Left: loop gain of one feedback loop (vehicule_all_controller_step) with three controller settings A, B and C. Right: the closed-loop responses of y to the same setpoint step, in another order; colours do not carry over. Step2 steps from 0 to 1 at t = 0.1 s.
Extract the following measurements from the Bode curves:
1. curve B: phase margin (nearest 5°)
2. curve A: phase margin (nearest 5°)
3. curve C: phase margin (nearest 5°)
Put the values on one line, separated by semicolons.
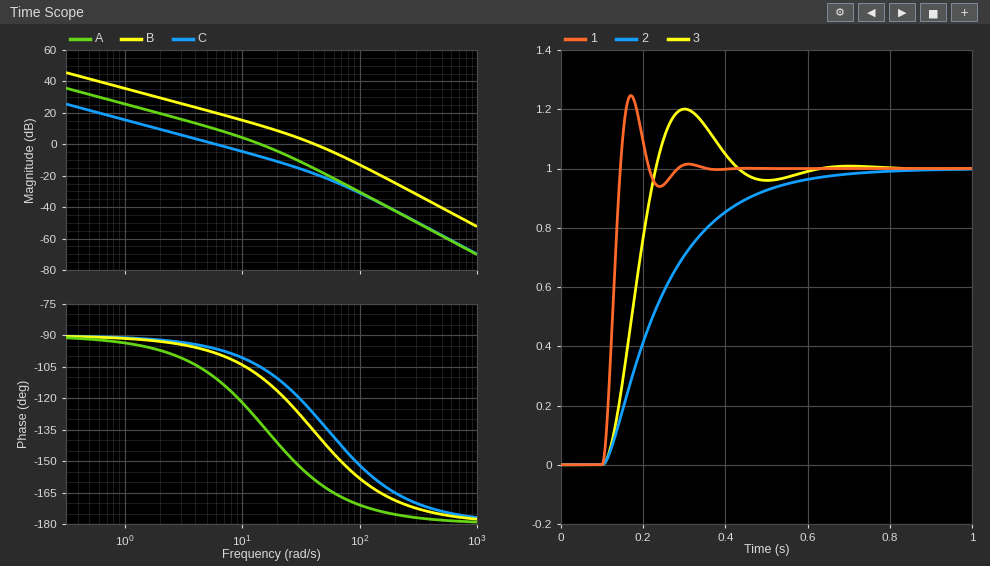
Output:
45°; 50°; 85°
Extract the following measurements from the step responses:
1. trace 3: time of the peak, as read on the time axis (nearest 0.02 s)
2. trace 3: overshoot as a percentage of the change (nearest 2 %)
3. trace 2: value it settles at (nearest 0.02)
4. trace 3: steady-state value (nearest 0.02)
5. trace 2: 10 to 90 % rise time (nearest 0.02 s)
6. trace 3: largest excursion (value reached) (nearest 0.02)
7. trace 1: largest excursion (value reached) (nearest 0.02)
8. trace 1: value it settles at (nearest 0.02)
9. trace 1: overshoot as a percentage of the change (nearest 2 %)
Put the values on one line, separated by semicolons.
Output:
0.30 s; 20 %; 1.00; 1.00; 0.32 s; 1.20; 1.24; 1.00; 24 %
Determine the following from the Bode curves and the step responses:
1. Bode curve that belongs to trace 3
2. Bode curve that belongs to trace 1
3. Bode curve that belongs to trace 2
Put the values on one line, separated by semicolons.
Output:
A; B; C
